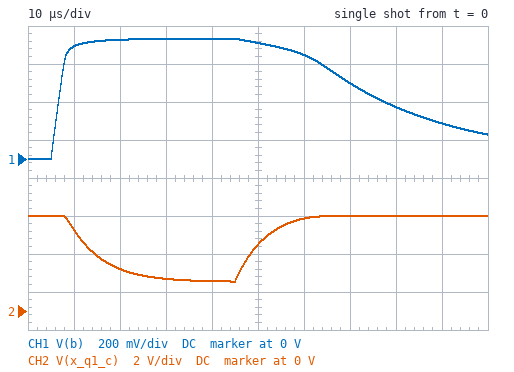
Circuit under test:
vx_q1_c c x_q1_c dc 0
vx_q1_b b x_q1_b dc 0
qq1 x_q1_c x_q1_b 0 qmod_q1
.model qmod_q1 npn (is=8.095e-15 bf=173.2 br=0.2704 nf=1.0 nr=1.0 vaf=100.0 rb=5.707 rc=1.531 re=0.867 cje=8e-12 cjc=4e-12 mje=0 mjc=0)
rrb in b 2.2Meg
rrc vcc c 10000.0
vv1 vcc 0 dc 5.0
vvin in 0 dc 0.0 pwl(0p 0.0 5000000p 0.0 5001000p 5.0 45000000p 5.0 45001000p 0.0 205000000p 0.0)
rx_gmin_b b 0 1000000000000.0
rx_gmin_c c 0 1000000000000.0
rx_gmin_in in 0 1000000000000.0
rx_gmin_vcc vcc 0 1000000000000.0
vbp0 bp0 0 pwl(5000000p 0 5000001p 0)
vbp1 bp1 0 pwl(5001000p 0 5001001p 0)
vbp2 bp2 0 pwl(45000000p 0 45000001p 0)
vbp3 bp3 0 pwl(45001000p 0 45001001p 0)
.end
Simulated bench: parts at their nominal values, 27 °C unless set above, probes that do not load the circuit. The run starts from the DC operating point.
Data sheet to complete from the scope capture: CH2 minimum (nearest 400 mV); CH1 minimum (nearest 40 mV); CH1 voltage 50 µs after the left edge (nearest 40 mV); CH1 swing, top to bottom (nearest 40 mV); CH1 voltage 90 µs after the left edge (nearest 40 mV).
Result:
1.6 V
0 V
600 mV
640 mV
200 mV
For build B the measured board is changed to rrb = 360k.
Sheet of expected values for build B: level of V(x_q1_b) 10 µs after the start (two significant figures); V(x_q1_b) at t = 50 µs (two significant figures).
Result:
640 mV
600 mV
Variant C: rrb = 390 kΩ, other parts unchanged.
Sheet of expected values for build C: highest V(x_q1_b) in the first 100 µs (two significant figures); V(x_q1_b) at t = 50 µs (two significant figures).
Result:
640 mV
600 mV
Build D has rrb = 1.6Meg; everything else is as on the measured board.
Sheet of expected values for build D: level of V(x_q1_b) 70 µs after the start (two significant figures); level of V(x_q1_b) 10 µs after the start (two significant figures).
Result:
350 mV
610 mV
